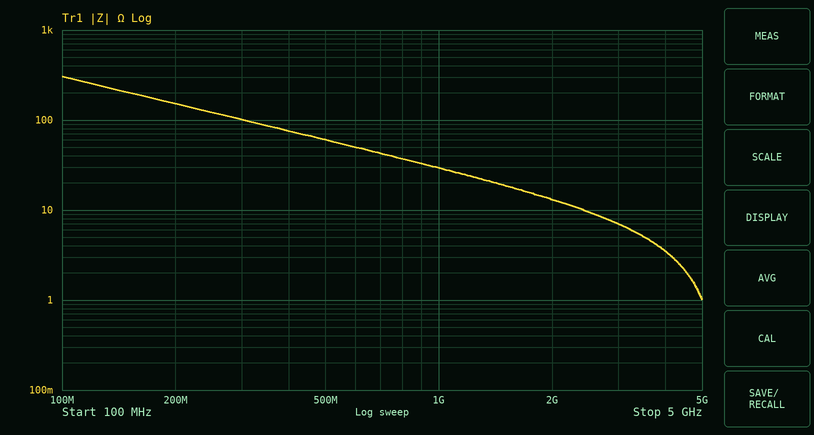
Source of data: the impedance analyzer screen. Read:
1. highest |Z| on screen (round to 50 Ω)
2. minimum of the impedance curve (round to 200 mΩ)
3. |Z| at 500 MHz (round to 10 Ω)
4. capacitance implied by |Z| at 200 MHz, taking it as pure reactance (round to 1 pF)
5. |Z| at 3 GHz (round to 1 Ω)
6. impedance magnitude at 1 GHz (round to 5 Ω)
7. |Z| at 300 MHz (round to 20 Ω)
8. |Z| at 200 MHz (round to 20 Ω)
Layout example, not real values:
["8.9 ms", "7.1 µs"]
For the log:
["300 Ω", "1.0 Ω", "60 Ω", "5 pF", "7 Ω", "30 Ω", "100 Ω", "160 Ω"]
